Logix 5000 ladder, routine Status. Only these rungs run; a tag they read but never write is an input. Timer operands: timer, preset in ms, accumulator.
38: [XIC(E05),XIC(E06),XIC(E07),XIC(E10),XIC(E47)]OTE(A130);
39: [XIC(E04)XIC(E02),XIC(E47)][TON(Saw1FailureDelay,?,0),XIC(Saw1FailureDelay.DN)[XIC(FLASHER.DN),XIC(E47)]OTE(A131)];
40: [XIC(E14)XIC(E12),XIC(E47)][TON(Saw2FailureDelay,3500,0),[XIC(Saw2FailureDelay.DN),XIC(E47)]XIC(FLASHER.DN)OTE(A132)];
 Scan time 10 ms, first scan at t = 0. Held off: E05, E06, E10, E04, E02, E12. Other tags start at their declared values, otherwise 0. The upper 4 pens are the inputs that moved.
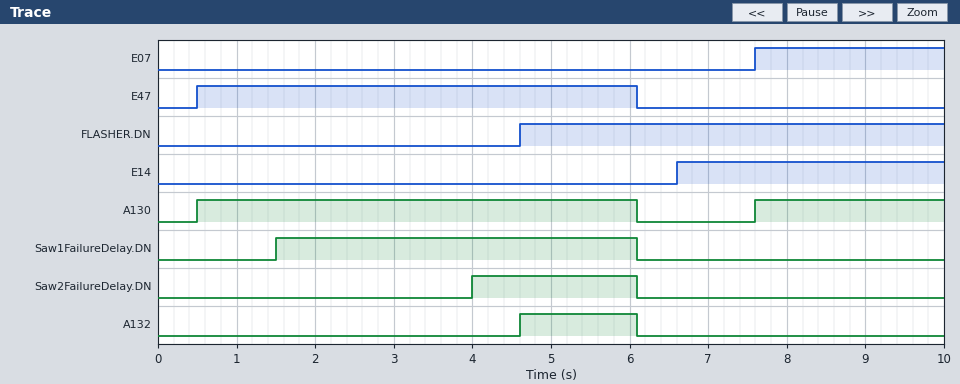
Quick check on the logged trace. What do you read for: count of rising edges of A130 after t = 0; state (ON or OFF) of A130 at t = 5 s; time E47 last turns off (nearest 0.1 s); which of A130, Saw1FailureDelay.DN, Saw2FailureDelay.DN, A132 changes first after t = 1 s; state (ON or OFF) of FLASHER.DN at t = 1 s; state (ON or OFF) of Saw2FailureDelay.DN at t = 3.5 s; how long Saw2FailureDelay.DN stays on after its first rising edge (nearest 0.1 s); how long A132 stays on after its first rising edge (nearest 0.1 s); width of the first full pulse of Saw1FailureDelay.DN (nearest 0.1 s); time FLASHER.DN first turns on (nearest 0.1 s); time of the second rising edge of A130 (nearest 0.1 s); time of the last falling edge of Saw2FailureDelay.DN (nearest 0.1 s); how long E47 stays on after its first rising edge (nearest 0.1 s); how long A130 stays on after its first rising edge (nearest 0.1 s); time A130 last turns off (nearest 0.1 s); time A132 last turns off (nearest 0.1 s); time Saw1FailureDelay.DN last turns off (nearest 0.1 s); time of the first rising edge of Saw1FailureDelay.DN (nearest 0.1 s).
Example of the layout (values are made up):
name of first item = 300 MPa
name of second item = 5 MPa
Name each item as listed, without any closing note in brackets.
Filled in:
count of rising edges of A130 after t = 0 = 2
state (ON or OFF) of A130 at t = 5 s = ON
time E47 last turns off = 6.1 s
which of A130, Saw1FailureDelay.DN, Saw2FailureDelay.DN, A132 changes first after t = 1 s = Saw1FailureDelay.DN
state (ON or OFF) of FLASHER.DN at t = 1 s = OFF
state (ON or OFF) of Saw2FailureDelay.DN at t = 3.5 s = OFF
how long Saw2FailureDelay.DN stays on after its first rising edge = 2.1 s
how long A132 stays on after its first rising edge = 1.5 s
width of the first full pulse of Saw1FailureDelay.DN = 4.6 s
time FLASHER.DN first turns on = 4.6 s
time of the second rising edge of A130 = 7.6 s
time of the last falling edge of Saw2FailureDelay.DN = 6.1 s
how long E47 stays on after its first rising edge = 5.6 s
how long A130 stays on after its first rising edge = 5.6 s
time A130 last turns off = 6.1 s
time A132 last turns off = 6.1 s
time Saw1FailureDelay.DN last turns off = 6.1 s
time of the first rising edge of Saw1FailureDelay.DN = 1.5 s
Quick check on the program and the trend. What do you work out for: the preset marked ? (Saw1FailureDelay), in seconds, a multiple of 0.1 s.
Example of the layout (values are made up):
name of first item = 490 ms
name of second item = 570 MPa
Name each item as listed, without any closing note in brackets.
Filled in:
the preset marked ? (Saw1FailureDelay), in seconds, a multiple of 0.1 s = 1.0 s
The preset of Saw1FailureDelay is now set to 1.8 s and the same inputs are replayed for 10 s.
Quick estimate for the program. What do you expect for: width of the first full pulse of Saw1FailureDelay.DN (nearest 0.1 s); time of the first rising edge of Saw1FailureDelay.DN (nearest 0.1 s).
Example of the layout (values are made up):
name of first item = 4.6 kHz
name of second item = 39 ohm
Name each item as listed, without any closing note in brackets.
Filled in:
width of the first full pulse of Saw1FailureDelay.DN = 3.8 s
time of the first rising edge of Saw1FailureDelay.DN = 2.3 s
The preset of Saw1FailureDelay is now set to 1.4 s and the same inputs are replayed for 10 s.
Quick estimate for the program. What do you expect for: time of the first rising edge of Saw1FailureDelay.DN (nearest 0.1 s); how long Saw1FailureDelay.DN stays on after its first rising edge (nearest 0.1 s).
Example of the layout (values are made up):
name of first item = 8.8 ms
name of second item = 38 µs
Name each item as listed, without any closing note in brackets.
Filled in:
time of the first rising edge of Saw1FailureDelay.DN = 1.9 s
how long Saw1FailureDelay.DN stays on after its first rising edge = 4.2 s
